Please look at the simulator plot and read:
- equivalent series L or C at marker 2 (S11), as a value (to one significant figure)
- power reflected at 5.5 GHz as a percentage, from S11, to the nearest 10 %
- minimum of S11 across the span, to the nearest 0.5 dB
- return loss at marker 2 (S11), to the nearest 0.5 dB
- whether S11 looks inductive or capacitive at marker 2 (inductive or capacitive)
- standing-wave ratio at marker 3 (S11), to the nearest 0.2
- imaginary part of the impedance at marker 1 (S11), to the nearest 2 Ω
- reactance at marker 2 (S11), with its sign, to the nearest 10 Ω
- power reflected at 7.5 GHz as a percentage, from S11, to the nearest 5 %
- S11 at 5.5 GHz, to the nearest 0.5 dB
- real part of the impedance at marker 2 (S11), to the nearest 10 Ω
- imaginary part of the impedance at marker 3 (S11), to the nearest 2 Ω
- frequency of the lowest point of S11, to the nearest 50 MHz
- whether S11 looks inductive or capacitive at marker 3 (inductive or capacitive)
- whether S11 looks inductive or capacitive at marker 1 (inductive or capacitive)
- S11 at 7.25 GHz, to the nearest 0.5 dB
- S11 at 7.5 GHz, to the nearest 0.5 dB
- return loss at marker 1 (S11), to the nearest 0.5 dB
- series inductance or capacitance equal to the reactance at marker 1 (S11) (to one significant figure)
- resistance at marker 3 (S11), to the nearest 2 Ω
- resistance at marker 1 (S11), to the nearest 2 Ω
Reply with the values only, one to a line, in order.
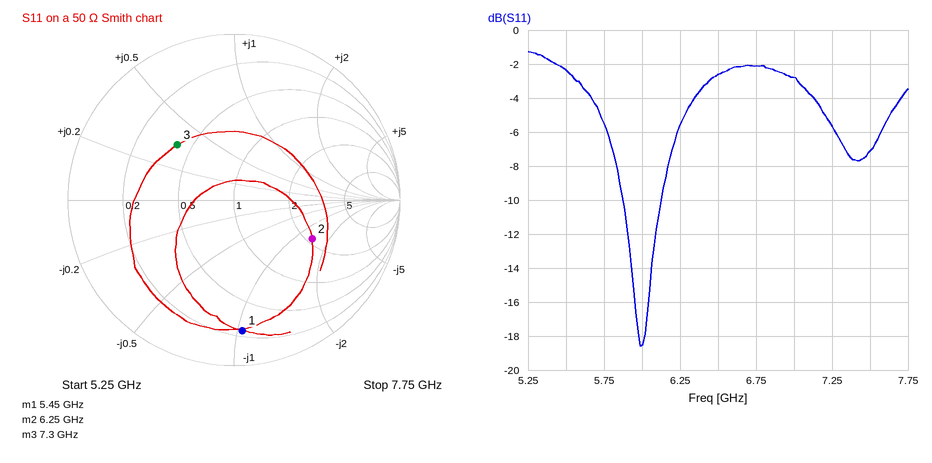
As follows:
400 fF
60 %
-18.5 dB
5.5 dB
capacitive
2.8
-52 Ω
-70 Ω
20 %
-2.5 dB
110 Ω
+18 Ω
6.00 GHz
inductive
capacitive
-5.5 dB
-7.0 dB
2.0 dB
600 fF
20 Ω
12 Ω
